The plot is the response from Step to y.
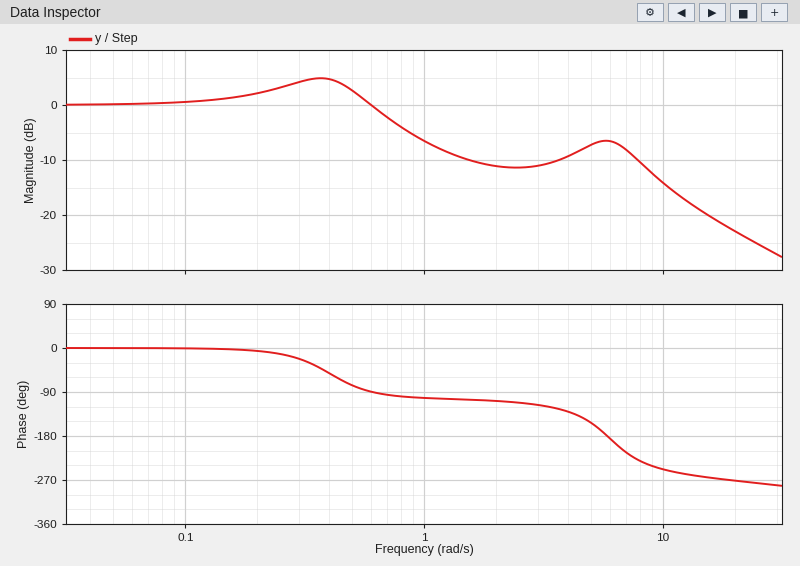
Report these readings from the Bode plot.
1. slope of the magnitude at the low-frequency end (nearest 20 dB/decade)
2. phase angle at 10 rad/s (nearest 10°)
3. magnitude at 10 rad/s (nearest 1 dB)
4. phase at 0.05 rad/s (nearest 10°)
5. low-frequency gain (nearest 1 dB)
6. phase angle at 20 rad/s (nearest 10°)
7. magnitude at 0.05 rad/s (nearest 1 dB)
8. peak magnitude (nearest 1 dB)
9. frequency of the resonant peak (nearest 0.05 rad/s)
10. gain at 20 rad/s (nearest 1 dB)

0 dB/decade
-250°
-14 dB
0°
0 dB
-270°
0 dB
5 dB
0.35 rad/s
-23 dB
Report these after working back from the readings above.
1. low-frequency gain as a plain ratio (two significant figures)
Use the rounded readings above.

1.0
